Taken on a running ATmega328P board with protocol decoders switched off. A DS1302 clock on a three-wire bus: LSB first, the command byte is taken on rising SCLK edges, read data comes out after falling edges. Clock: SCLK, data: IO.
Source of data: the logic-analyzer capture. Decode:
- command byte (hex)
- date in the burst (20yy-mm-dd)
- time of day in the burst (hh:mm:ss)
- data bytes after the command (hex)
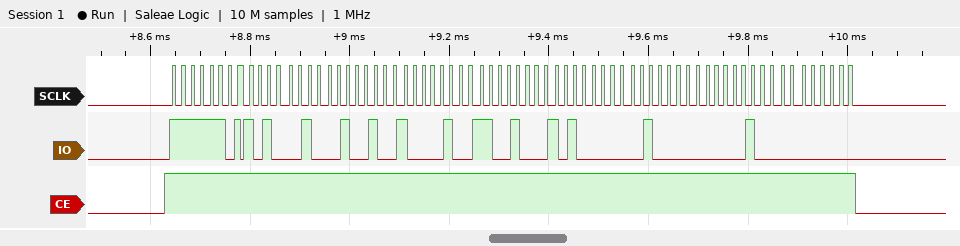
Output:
0xBF
2020-05-13
21:24:45
45 24 21 13 05 04 20 00
